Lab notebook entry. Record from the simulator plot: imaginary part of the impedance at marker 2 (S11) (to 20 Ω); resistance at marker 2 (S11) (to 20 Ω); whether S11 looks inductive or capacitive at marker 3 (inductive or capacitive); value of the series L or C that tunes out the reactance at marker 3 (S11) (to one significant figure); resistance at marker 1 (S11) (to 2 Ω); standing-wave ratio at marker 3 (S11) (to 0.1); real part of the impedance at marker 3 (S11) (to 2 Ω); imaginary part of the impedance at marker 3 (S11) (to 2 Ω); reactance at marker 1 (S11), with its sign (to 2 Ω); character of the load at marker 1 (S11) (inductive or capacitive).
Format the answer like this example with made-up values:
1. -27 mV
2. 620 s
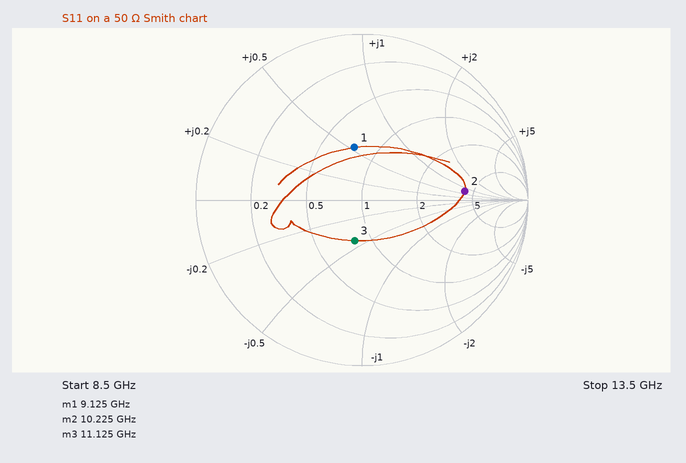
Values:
1. +40 Ω
2. 200 Ω
3. capacitive
4. 300 pH
5. 38 Ω
6. 1.7
7. 40 Ω
8. -22 Ω
9. +26 Ω
10. inductive
